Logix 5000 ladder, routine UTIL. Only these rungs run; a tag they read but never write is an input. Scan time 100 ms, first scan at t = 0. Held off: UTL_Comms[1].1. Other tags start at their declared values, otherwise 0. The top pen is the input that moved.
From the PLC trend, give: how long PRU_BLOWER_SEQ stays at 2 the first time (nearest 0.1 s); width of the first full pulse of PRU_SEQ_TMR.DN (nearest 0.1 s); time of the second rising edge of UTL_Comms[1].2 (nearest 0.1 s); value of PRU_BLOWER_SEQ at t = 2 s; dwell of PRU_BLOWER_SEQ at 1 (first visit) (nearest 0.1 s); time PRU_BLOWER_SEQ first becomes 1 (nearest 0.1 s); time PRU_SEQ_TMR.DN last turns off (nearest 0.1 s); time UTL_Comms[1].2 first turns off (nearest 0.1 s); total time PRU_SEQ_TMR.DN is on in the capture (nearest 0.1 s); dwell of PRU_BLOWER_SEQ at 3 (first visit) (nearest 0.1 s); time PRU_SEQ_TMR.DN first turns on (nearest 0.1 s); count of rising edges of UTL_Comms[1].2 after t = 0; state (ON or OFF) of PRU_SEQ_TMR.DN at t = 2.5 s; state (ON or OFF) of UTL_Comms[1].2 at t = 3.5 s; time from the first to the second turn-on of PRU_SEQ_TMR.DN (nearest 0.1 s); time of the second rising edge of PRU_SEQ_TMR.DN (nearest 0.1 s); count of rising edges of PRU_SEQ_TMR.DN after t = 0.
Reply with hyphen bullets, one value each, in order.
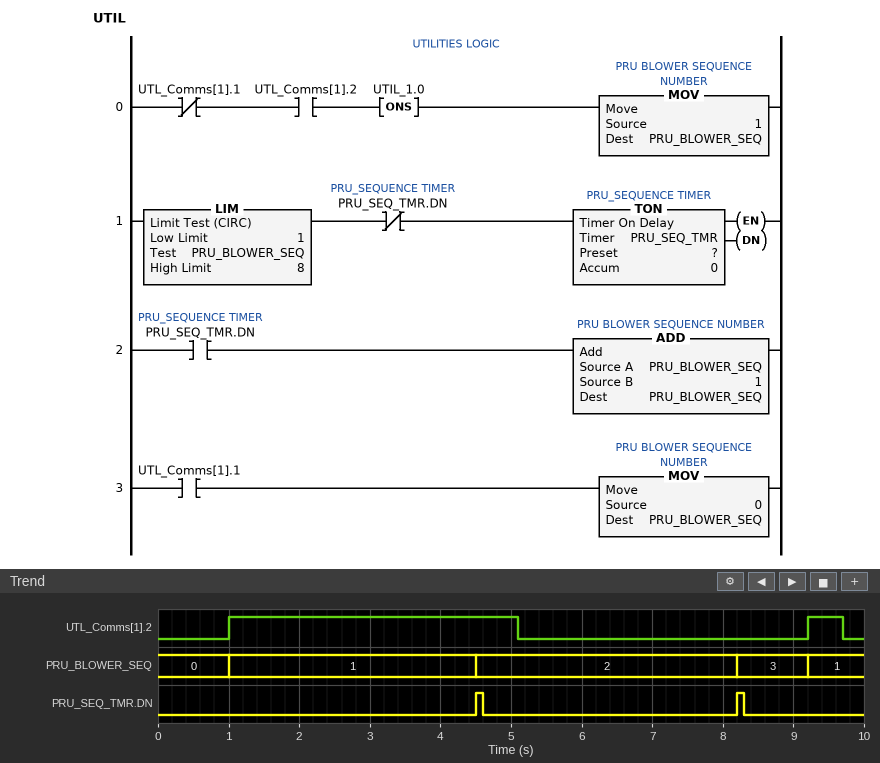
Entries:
- 3.7 s
- 0.1 s
- 9.2 s
- 1
- 3.5 s
- 1.0 s
- 8.3 s
- 5.1 s
- 0.2 s
- 1.0 s
- 4.5 s
- 2
- OFF
- ON
- 3.7 s
- 8.2 s
- 2
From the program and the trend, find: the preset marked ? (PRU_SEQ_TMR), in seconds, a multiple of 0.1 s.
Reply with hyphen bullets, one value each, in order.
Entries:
- 3.5 s
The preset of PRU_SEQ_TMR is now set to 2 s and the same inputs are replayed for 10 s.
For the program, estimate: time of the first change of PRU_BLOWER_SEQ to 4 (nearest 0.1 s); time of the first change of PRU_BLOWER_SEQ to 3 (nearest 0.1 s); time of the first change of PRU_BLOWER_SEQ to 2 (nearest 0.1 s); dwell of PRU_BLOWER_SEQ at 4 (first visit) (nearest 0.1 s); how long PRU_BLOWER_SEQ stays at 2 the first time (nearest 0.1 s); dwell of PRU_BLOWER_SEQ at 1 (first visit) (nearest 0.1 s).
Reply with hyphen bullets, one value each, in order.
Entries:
- 7.4 s
- 5.2 s
- 3.0 s
- 1.8 s
- 2.2 s
- 2.0 s
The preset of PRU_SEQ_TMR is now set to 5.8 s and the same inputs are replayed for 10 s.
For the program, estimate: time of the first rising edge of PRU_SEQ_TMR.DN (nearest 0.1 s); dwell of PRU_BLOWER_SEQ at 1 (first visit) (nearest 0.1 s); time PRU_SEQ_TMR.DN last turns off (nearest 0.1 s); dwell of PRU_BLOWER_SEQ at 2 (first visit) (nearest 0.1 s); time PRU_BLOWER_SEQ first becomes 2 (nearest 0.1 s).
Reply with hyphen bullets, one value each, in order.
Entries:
- 6.8 s
- 5.8 s
- 6.9 s
- 2.4 s
- 6.8 s
